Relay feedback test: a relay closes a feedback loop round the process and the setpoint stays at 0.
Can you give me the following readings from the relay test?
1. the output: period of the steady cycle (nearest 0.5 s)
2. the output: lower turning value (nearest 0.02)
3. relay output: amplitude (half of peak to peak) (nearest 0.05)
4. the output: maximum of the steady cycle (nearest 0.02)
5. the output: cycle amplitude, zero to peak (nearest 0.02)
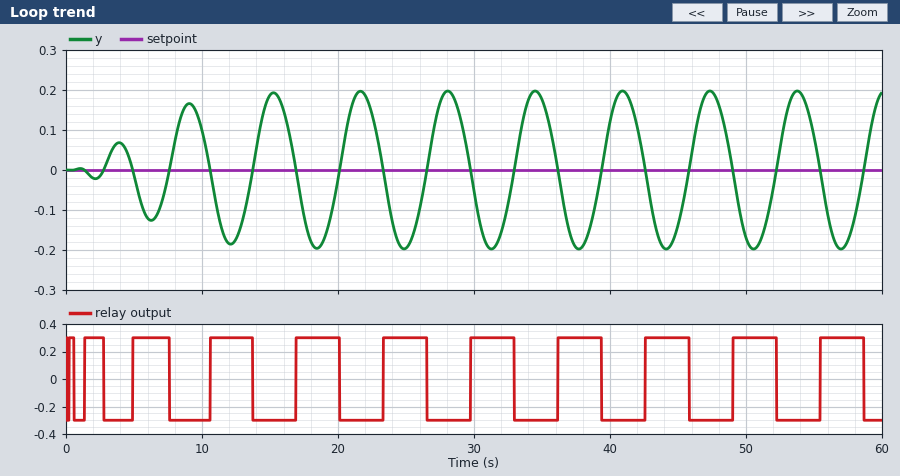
6.5 s
-0.20
0.30
0.20
0.20
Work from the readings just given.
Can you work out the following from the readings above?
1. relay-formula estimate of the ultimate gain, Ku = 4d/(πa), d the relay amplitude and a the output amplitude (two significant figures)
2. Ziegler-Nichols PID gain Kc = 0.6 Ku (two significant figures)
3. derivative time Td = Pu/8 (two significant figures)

1.9
1.1
0.81 s
